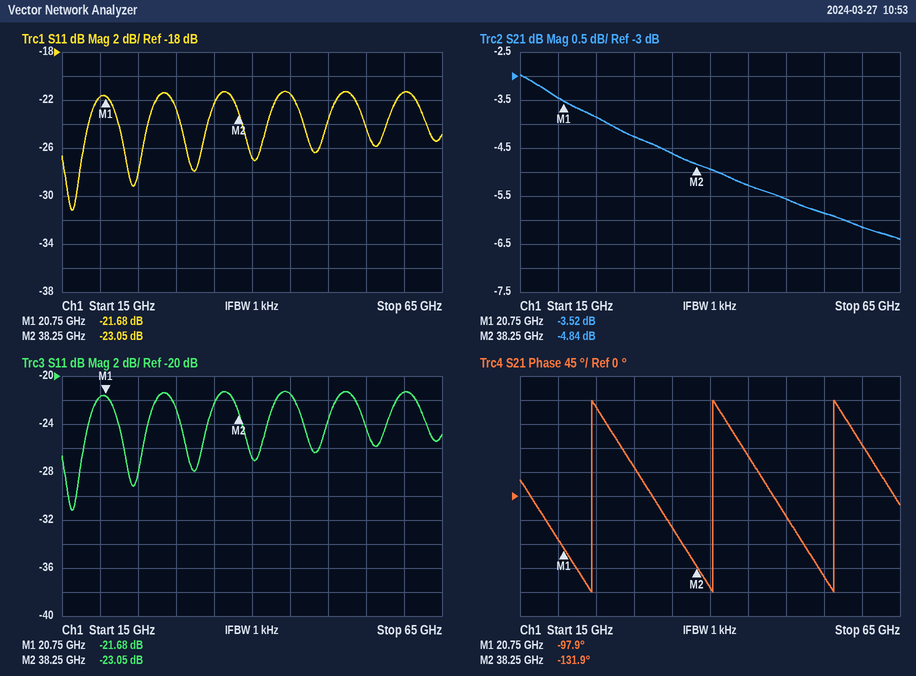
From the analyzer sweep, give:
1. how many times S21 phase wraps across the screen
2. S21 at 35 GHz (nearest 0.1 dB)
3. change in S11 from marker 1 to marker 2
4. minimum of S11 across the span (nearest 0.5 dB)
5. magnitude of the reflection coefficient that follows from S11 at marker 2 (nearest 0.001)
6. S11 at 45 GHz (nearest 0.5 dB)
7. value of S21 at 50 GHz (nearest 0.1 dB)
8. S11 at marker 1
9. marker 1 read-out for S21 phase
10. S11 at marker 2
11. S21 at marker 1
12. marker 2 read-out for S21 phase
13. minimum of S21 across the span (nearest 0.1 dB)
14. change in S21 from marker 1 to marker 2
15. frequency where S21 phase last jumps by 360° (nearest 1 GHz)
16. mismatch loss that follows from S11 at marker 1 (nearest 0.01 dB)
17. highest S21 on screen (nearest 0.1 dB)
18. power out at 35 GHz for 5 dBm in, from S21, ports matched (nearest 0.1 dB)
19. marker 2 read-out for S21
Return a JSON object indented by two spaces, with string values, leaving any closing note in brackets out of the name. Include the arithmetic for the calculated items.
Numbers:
{
  "how many times S21 phase wraps across the screen": "3",
  "S21 at 35 GHz": "-4.6 dB",
  "change in S11 from marker 1 to marker 2": "-23.05 − (-21.68) = -1.37 dB",
  "minimum of S11 across the span": "-31.0 dB",
  "magnitude of the reflection coefficient that follows from S11 at marker 2": "10^(-23.05/20) ≈ 0.070",
  "S11 at 45 GHz": "-21.5 dB",
  "value of S21 at 50 GHz": "-5.6 dB",
  "S11 at marker 1": "-21.68 dB",
  "marker 1 read-out for S21 phase": "-97.9°",
  "S11 at marker 2": "-23.05 dB",
  "S21 at marker 1": "-3.52 dB",
  "marker 2 read-out for S21 phase": "-131.9°",
  "minimum of S21 across the span": "-6.4 dB",
  "change in S21 from marker 1 to marker 2": "-4.84 − (-3.52) = -1.32 dB",
  "frequency where S21 phase last jumps by 360°": "56 GHz",
  "mismatch loss that follows from S11 at marker 1": "−10 log10(1 − 10^(-21.68/10)) ≈ 0.03 dB",
  "highest S21 on screen": "-3.0 dB",
  "power out at 35 GHz for 5 dBm in, from S21, ports matched": "5 dBm + (-4.6 dB) = 0.4 dBm",
  "marker 2 read-out for S21": "-4.84 dB"
}
